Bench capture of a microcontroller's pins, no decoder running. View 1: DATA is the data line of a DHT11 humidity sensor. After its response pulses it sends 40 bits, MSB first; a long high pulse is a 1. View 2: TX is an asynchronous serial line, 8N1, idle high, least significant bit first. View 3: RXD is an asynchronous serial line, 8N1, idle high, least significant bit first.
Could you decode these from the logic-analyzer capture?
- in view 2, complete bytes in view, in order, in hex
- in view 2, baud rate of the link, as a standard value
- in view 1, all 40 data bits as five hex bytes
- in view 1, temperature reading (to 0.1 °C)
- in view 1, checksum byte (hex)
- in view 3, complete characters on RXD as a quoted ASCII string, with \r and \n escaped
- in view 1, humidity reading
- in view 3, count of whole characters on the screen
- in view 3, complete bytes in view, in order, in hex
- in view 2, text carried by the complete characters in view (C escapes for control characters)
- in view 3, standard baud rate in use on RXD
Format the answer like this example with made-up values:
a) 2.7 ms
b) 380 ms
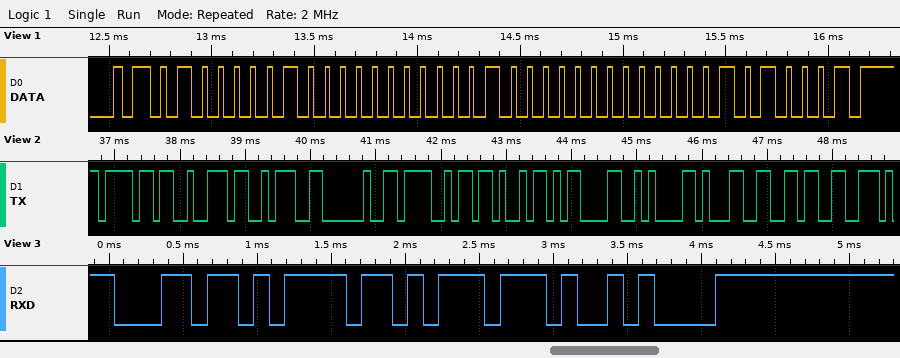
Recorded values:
a) 6F 72 3A 20 4F 4B 0D 0A 31 36
b) 9600 baud
c) 41 00 10 00 51
d) 16.0 °C
e) 0x51
f) "low\n"
g) 65 %
h) 4
i) 6C 6F 77 0A
j) "or: OK\r\n16"
k) 9600 baud
